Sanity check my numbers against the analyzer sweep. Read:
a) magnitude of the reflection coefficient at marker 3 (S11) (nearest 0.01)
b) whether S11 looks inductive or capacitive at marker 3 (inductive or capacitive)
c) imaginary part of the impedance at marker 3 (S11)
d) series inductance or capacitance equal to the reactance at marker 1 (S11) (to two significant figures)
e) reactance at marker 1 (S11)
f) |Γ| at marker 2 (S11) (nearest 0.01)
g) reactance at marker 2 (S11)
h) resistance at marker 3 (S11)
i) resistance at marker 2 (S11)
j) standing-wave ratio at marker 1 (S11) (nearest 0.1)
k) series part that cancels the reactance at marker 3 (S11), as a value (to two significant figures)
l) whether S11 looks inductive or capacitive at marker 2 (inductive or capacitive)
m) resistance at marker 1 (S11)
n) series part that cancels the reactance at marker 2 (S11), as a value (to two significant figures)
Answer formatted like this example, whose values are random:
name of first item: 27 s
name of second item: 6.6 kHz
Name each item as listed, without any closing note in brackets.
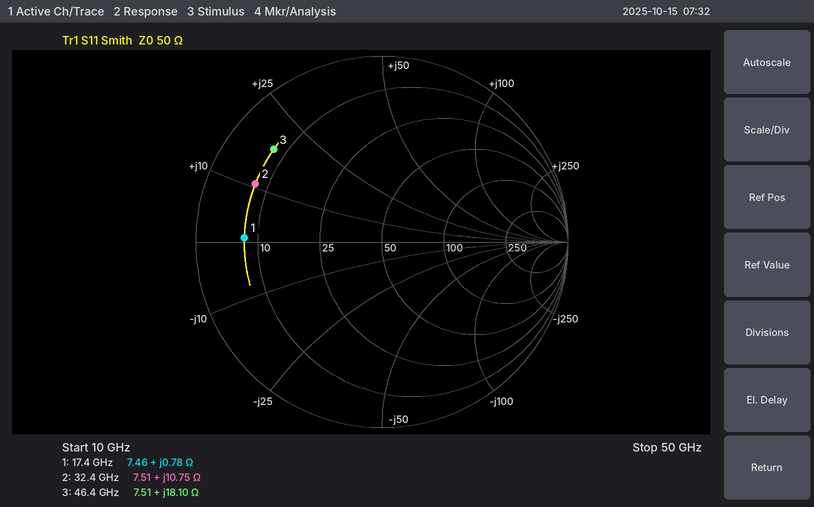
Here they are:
magnitude of the reflection coefficient at marker 3 (S11): 0.77
whether S11 looks inductive or capacitive at marker 3: inductive
imaginary part of the impedance at marker 3: +18.10 Ω
series inductance or capacitance equal to the reactance at marker 1 (S11): 7.1 pH
reactance at marker 1: +0.78 Ω
|Γ| at marker 2 (S11): 0.75
reactance at marker 2: +10.75 Ω
resistance at marker 3: 7.51 Ω
resistance at marker 2: 7.51 Ω
standing-wave ratio at marker 1 (S11): 6.7
series part that cancels the reactance at marker 3 (S11), as a value: 190 fF
whether S11 looks inductive or capacitive at marker 2: inductive
resistance at marker 1: 7.46 Ω
series part that cancels the reactance at marker 2 (S11), as a value: 460 fF
